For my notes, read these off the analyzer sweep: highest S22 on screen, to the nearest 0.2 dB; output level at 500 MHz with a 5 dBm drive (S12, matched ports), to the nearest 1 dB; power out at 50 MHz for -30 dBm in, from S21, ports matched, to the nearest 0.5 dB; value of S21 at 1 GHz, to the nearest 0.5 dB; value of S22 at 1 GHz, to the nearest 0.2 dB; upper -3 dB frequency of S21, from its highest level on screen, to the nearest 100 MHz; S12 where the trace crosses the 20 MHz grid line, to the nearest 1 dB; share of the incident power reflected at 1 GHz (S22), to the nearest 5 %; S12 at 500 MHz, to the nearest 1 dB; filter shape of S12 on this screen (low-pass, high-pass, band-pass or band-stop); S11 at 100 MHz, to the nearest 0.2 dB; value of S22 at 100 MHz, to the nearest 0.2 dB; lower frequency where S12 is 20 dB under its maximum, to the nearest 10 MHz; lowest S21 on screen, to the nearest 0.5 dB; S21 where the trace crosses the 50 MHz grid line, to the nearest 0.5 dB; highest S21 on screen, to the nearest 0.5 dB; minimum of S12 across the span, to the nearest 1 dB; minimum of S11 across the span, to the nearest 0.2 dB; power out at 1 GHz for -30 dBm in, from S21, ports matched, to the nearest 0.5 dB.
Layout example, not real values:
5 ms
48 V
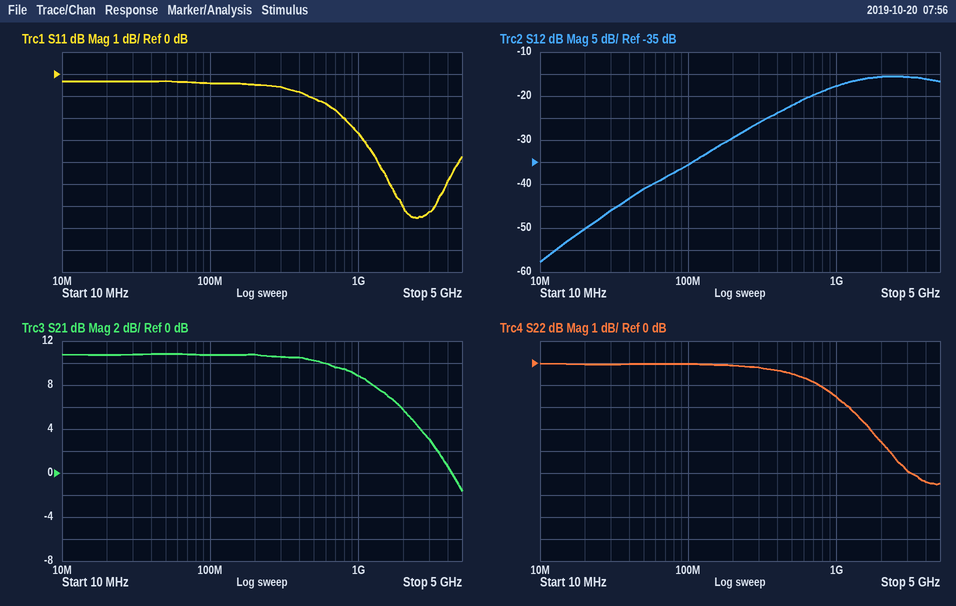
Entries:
0.0 dB
-17 dBm
-19.0 dBm
9.0 dB
-1.6 dB
1.3 GHz
-50 dB
70 %
-22 dB
high-pass
-0.4 dB
0.0 dB
100 MHz
-1.5 dB
11.0 dB
11.0 dB
-58 dB
-6.6 dB
-21.0 dBm
